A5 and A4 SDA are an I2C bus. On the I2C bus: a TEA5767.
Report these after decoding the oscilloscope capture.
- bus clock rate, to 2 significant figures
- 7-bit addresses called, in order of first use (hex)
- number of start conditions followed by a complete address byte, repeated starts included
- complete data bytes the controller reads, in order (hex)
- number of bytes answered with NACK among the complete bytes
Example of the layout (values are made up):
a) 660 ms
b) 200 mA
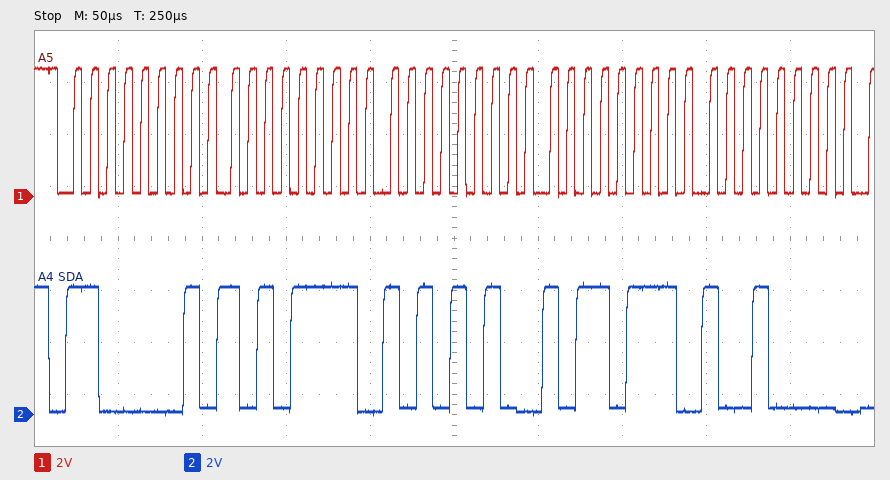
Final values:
a) 100 kHz
b) 0x60
c) 1
d) AF AA B7 90
e) 0
